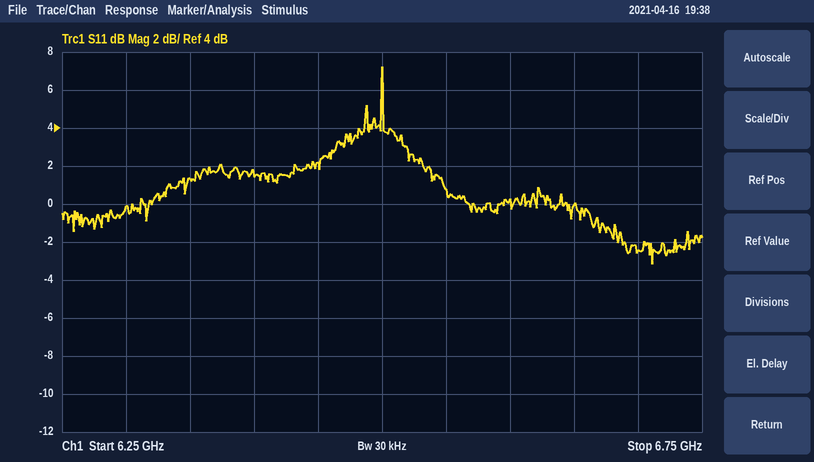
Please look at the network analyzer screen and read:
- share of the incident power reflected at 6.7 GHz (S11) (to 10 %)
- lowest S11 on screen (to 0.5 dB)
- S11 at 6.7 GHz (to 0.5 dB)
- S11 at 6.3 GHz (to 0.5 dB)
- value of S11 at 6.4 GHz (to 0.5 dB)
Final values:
60 %
-3.0 dB
-2.5 dB
0.0 dB
1.5 dB
